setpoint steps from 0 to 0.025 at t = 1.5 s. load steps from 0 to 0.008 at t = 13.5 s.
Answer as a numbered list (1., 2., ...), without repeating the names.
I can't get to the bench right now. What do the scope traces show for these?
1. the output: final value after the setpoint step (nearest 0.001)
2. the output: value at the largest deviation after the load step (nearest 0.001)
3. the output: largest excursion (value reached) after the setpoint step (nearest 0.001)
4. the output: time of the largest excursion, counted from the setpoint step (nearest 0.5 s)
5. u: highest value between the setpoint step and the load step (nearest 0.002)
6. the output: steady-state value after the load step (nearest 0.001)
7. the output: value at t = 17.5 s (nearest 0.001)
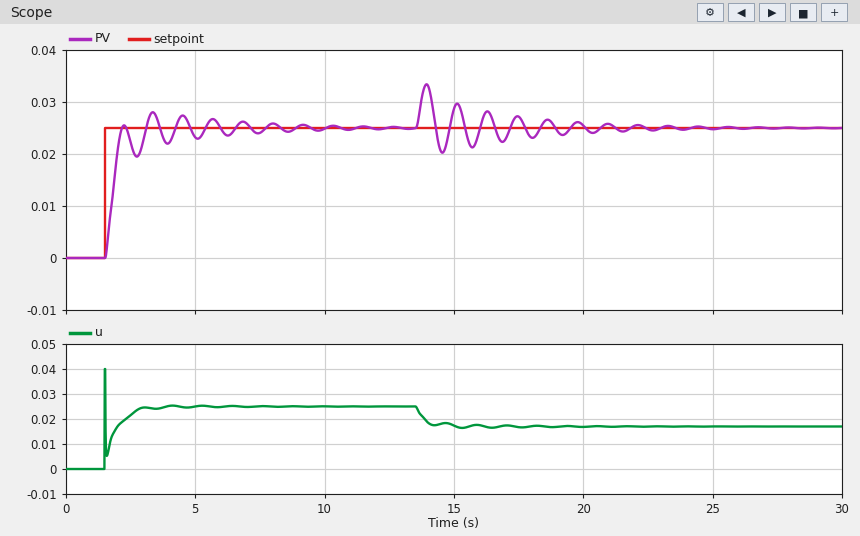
1. 0.025
2. 0.033
3. 0.028
4. 2.0 s
5. 0.040
6. 0.025
7. 0.027
